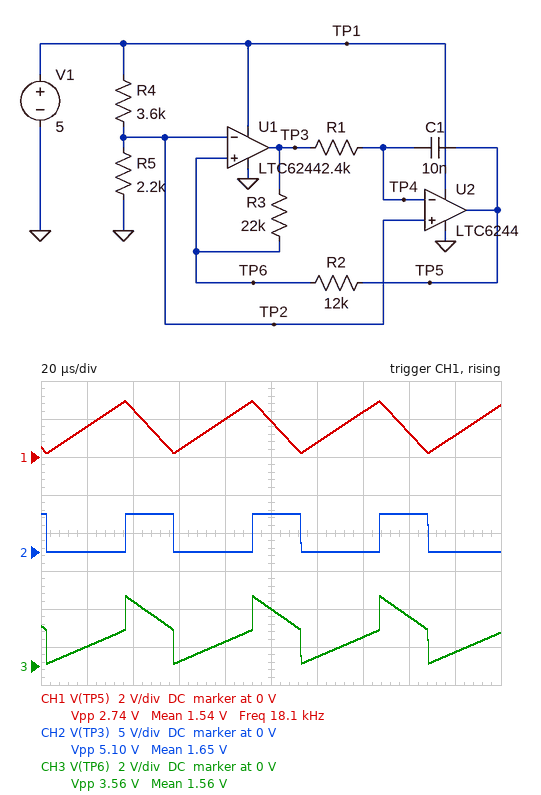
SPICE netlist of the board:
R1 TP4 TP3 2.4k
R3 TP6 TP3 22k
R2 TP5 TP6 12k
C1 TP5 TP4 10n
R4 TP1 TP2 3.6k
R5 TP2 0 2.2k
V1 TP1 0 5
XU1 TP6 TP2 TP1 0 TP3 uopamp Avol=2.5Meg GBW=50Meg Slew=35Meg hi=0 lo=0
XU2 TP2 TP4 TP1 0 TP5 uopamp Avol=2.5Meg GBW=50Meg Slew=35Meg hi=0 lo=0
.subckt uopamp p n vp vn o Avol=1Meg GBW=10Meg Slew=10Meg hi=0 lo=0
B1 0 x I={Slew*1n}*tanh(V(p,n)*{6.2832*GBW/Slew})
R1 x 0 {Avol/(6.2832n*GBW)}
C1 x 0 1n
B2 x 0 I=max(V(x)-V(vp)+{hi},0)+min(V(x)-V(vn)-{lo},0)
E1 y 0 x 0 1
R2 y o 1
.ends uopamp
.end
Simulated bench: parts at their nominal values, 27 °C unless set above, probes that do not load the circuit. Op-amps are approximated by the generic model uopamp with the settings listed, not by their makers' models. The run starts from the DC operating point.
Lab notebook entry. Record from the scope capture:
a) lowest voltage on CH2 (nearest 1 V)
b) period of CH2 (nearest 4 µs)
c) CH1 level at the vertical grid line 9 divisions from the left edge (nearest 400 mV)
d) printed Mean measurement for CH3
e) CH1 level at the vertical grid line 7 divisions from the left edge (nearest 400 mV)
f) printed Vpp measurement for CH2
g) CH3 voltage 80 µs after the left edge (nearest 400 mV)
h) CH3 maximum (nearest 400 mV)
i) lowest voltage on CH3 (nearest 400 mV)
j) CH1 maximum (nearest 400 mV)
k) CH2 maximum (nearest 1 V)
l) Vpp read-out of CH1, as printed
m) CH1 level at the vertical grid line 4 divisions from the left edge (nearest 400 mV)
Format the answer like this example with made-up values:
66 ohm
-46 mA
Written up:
0 V
56 µs
1.2 V
1.56 V
2.4 V
5.10 V
1.2 V
3.6 V
0 V
2.8 V
5 V
2.74 V
2.0 V
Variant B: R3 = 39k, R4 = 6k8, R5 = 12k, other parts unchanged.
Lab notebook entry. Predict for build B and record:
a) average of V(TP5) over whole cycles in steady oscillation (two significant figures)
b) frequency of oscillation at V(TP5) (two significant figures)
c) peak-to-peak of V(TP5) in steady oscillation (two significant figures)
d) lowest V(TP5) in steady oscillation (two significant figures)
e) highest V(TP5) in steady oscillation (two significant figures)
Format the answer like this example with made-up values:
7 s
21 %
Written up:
3.4 V
31 kHz
1.6 V
2.6 V
4.2 V
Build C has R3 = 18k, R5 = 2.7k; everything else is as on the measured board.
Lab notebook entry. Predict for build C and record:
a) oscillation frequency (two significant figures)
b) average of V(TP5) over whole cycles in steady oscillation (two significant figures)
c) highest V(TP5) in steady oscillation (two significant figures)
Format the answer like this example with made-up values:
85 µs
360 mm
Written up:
15 kHz
1.9 V
3.6 V
